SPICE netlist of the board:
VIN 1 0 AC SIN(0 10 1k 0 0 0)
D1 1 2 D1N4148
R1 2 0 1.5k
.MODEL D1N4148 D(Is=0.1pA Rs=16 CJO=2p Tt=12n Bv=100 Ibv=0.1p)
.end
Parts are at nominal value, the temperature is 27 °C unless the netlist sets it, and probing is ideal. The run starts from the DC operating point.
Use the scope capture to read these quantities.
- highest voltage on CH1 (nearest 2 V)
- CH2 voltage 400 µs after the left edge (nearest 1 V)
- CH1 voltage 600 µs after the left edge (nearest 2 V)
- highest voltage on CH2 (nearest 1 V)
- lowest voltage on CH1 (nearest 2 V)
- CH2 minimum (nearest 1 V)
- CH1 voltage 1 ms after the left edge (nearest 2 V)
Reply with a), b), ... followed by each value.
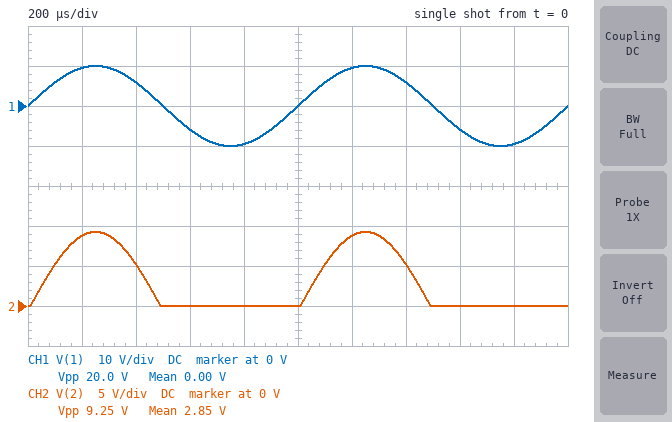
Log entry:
a) 10 V
b) 5 V
c) -6 V
d) 9 V
e) -10 V
f) 0 V
g) 0 V
